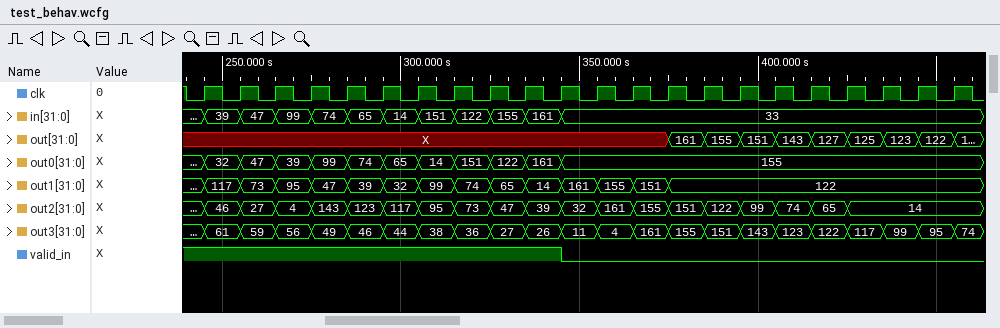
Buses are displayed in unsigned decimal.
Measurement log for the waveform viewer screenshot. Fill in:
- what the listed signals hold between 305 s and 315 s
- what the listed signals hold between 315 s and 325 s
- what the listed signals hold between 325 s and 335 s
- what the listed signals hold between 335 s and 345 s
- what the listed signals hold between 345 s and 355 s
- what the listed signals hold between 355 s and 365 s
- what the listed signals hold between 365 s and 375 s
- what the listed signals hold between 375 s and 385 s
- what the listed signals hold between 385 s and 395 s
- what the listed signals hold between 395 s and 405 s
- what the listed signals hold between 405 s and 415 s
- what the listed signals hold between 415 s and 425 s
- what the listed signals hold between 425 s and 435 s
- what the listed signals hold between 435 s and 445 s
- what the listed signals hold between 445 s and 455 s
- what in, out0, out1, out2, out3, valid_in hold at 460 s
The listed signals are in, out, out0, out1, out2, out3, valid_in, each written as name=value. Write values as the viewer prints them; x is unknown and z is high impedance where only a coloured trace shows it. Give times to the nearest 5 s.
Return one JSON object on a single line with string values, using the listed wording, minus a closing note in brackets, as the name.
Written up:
{"what the listed signals hold between 305 s and 315 s": "in=151, out=X, out0=14, out1=99, out2=95, out3=38, valid_in=1", "what the listed signals hold between 315 s and 325 s": "in=122, out=X, out0=151, out1=74, out2=73, out3=36, valid_in=1", "what the listed signals hold between 325 s and 335 s": "in=155, out=X, out0=122, out1=65, out2=47, out3=27, valid_in=1", "what the listed signals hold between 335 s and 345 s": "in=161, out=X, out0=161, out1=14, out2=39, out3=26, valid_in=1", "what the listed signals hold between 345 s and 355 s": "in=33, out=X, out0=155, out1=161, out2=32, out3=11, valid_in=0", "what the listed signals hold between 355 s and 365 s": "in=33, out=X, out0=155, out1=155, out2=161, out3=4, valid_in=0", "what the listed signals hold between 365 s and 375 s": "in=33, out=X, out0=155, out1=151, out2=155, out3=161, valid_in=0", "what the listed signals hold between 375 s and 385 s": "in=33, out=161, out0=155, out1=122, out2=151, out3=155, valid_in=0", "what the listed signals hold between 385 s and 395 s": "in=33, out=155, out0=155, out1=122, out2=122, out3=151, valid_in=0", "what the listed signals hold between 395 s and 405 s": "in=33, out=151, out0=155, out1=122, out2=99, out3=143, valid_in=0", "what the listed signals hold between 405 s and 415 s": "in=33, out=143, out0=155, out1=122, out2=74, out3=123, valid_in=0", "what the listed signals hold between 415 s and 425 s": "in=33, out=127, out0=155, out1=122, out2=65, out3=122, valid_in=0", "what the listed signals hold between 425 s and 435 s": "in=33, out=125, out0=155, out1=122, out2=14, out3=117, valid_in=0", "what the listed signals hold between 435 s and 445 s": "in=33, out=123, out0=155, out1=122, out2=14, out3=99, valid_in=0", "what the listed signals hold between 445 s and 455 s": "in=33, out=122, out0=155, out1=122, out2=14, out3=95, valid_in=0", "what in, out0, out1, out2, out3, valid_in hold at 460 s": "in=33, out0=155, out1=122, out2=14, out3=74, valid_in=0"}
